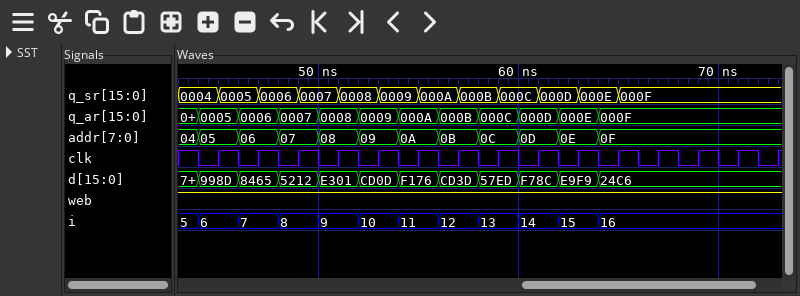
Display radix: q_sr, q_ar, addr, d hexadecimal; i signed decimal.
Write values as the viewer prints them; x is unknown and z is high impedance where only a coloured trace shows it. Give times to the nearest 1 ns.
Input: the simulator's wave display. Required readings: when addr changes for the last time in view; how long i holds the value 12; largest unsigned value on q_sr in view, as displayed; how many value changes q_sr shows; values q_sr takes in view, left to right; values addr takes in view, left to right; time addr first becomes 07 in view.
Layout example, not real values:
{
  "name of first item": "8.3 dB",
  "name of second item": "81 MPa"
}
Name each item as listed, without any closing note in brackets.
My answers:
{
  "when addr changes for the last time in view": "64 ns",
  "how long i holds the value 12": "2 ns",
  "largest unsigned value on q_sr in view, as displayed": "000F",
  "how many value changes q_sr shows": "11",
  "values q_sr takes in view, left to right": "0004, 0005, 0006, 0007, 0008, 0009, 000A, 000B, 000C, 000D, 000E, 000F",
  "values addr takes in view, left to right": "04, 05, 06, 07, 08, 09, 0A, 0B, 0C, 0D, 0E, 0F",
  "time addr first becomes 07 in view": "48 ns"
}
